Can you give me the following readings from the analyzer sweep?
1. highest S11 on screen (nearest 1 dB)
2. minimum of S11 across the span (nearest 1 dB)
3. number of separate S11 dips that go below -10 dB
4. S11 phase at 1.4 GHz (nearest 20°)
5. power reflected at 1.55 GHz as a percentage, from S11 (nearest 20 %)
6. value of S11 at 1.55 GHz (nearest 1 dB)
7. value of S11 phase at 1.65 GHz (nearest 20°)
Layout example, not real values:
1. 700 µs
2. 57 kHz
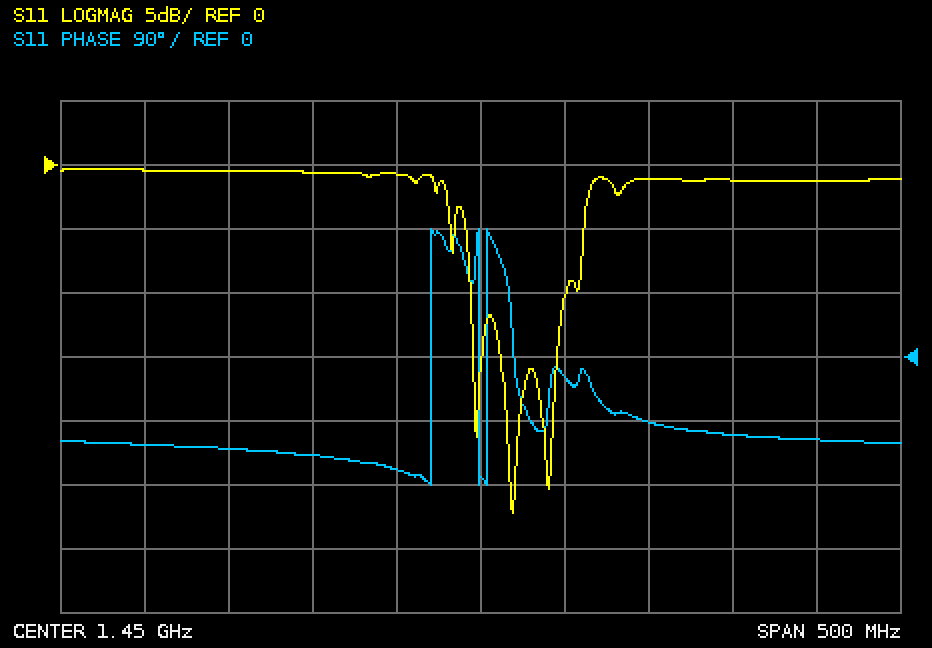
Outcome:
1. 0 dB
2. -27 dB
3. 3
4. -160°
5. 80 %
6. -1 dB
7. -120°
